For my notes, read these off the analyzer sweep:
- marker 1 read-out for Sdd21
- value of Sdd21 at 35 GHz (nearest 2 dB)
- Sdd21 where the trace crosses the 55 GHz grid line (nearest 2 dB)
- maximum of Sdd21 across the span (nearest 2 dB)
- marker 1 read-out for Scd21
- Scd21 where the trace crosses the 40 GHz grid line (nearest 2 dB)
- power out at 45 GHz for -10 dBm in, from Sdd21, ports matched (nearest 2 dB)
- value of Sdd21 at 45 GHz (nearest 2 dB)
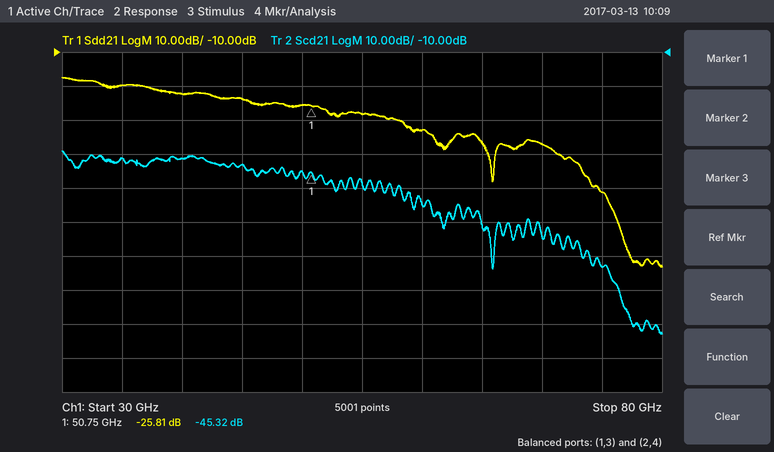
-25.81 dB
-20 dB
-28 dB
-18 dB
-45.32 dB
-42 dB
-34 dBm
-24 dB
